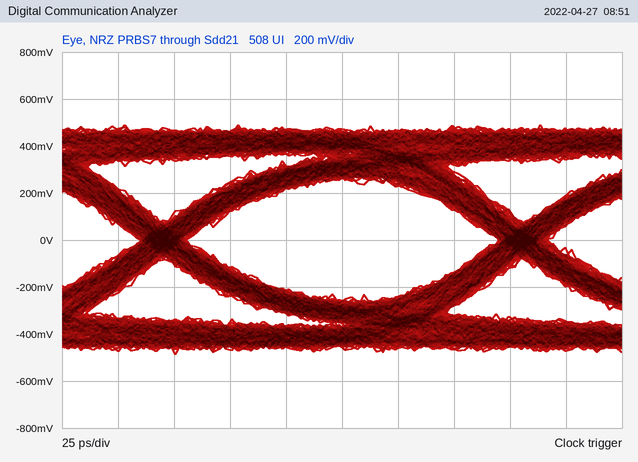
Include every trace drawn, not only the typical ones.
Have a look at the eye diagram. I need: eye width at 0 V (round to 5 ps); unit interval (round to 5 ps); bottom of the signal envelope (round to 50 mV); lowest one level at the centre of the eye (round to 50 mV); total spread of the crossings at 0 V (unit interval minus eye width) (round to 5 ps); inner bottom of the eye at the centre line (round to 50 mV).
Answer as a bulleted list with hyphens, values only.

- 140 ps
- 160 ps
- -500 mV
- 250 mV
- 20 ps
- -250 mV
